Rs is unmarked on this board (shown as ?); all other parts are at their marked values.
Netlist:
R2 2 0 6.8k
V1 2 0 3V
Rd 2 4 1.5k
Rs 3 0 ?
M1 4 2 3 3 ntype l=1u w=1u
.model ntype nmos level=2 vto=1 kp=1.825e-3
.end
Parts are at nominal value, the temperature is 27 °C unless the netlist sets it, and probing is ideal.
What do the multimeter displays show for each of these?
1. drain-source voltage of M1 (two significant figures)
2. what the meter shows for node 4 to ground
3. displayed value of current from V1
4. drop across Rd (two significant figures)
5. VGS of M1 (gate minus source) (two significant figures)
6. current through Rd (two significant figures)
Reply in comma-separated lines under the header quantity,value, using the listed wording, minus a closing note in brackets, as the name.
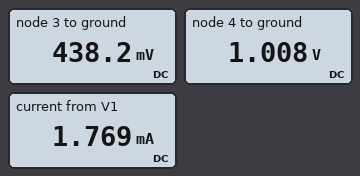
quantity,value
drain-source voltage of M1,570 mV
what the meter shows for node 4 to ground,1.008 V
displayed value of current from V1,1.769 mA
drop across Rd,2.0 V
VGS of M1 (gate minus source),2.6 V
current through Rd,1.3 mA
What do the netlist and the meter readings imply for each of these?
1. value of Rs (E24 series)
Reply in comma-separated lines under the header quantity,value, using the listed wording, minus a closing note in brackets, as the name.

quantity,value
value of Rs,330 Ω
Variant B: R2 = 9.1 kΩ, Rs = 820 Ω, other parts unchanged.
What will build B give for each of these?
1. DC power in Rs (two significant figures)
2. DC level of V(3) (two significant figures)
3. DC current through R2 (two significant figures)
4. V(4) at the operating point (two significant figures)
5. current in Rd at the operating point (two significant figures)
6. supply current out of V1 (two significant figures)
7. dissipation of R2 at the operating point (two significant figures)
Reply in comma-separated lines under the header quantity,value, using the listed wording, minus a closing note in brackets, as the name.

quantity,value
DC power in Rs,840 µW
DC level of V(3),830 mV
DC current through R2,330 µA
V(4) at the operating point,1.5 V
current in Rd at the operating point,1.0 mA
supply current out of V1,1.3 mA
dissipation of R2 at the operating point,990 µW
